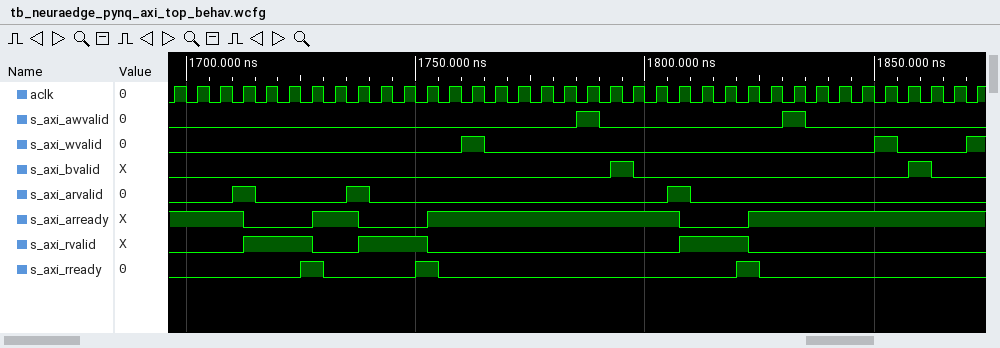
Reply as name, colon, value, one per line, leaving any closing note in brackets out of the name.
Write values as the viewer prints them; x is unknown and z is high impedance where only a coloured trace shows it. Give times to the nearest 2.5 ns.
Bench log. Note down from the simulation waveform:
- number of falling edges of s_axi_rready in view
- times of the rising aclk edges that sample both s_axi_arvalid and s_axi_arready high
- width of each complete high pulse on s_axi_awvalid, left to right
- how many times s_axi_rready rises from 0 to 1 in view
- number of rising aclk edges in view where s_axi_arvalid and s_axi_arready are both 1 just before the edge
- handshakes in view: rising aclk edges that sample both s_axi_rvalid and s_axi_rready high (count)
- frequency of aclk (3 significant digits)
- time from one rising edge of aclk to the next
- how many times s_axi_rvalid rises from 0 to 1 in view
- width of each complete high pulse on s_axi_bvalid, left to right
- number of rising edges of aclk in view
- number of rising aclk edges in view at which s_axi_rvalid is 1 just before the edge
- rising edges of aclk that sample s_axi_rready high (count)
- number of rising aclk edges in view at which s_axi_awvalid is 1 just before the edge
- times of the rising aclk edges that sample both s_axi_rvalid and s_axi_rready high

number of falling edges of s_axi_rready in view: 3
times of the rising aclk edges that sample both s_axi_arvalid and s_axi_arready high: 1712.5 ns, 1737.5 ns, 1807.5 ns
width of each complete high pulse on s_axi_awvalid, left to right: 5 ns, 5 ns
how many times s_axi_rready rises from 0 to 1 in view: 3
number of rising aclk edges in view where s_axi_arvalid and s_axi_arready are both 1 just before the edge: 3
handshakes in view: rising aclk edges that sample both s_axi_rvalid and s_axi_rready high: 3
frequency of aclk: 200 MHz
time from one rising edge of aclk to the next: 5 ns
how many times s_axi_rvalid rises from 0 to 1 in view: 3
width of each complete high pulse on s_axi_bvalid, left to right: 5 ns, 5 ns
number of rising edges of aclk in view: 36
number of rising aclk edges in view at which s_axi_rvalid is 1 just before the edge: 9
rising edges of aclk that sample s_axi_rready high: 3
number of rising aclk edges in view at which s_axi_awvalid is 1 just before the edge: 2
times of the rising aclk edges that sample both s_axi_rvalid and s_axi_rready high: 1727.5 ns, 1752.5 ns, 1822.5 ns
